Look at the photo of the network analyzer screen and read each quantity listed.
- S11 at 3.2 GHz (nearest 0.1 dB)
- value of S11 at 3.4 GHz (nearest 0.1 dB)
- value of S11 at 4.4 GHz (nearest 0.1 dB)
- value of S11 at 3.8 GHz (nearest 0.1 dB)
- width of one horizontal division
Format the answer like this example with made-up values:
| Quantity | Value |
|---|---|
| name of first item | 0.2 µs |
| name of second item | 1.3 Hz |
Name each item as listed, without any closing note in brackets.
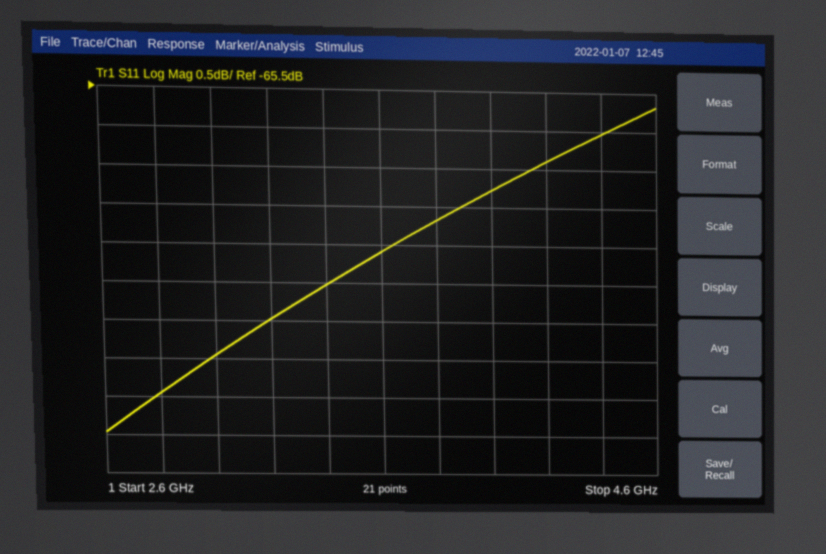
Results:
| Quantity | Value |
|---|---|
| S11 at 3.2 GHz | -68.5 dB |
| value of S11 at 3.4 GHz | -68.0 dB |
| value of S11 at 4.4 GHz | -66.0 dB |
| value of S11 at 3.8 GHz | -67.2 dB |
| width of one horizontal division | 200 MHz |
